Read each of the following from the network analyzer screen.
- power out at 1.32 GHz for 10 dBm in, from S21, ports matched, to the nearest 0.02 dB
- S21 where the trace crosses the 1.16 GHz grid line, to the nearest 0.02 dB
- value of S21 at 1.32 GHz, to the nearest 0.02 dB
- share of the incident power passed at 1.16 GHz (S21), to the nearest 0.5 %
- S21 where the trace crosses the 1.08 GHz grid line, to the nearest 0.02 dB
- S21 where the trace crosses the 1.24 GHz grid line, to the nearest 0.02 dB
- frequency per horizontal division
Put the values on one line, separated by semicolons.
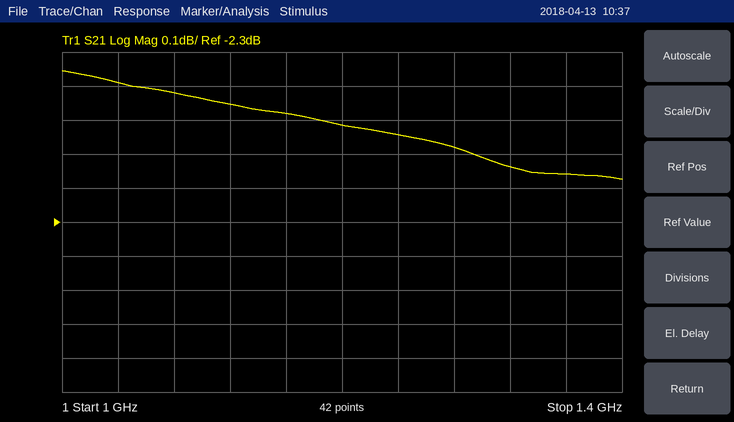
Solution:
7.86 dBm; -1.98 dB; -2.14 dB; 63.5 %; -1.92 dB; -2.04 dB; 40 MHz
